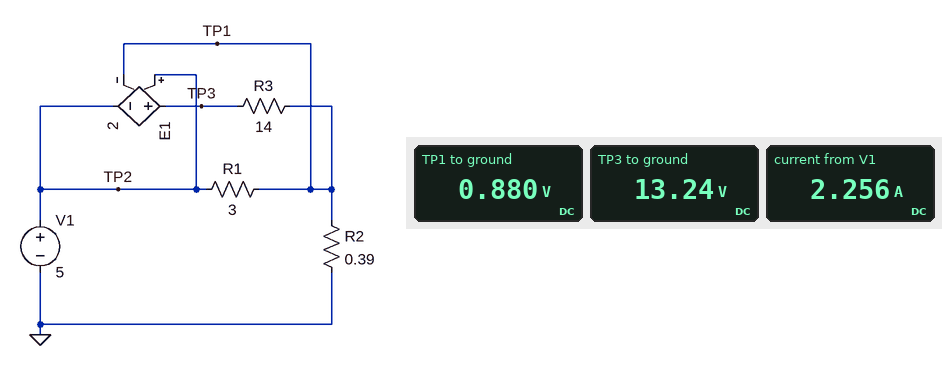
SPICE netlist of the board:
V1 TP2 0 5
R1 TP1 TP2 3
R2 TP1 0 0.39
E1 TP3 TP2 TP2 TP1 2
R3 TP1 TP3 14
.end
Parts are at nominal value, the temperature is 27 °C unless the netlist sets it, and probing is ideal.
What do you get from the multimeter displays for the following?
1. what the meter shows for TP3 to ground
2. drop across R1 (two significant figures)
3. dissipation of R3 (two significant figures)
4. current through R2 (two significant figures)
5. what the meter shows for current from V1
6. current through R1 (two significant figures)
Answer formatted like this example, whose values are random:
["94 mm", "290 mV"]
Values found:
["13.24 V", "4.1 V", "11 W", "2.3 A", "2.256 A", "1.4 A"]
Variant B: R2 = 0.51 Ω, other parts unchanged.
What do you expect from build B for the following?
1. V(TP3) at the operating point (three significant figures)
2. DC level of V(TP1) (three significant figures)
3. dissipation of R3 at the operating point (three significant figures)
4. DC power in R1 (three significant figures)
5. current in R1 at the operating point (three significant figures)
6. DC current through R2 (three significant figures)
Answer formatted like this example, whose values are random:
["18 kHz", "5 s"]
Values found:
["12.8 V", "1.09 V", "9.82 W", "5.09 W", "1.30 A", "2.14 A"]
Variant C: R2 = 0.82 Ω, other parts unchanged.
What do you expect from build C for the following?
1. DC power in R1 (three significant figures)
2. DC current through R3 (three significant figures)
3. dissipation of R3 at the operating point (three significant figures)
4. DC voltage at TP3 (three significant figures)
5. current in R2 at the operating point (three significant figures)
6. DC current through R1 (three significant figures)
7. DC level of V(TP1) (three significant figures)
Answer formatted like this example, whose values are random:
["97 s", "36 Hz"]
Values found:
["3.97 W", "739 mA", "7.65 W", "11.9 V", "1.89 A", "1.15 A", "1.55 V"]
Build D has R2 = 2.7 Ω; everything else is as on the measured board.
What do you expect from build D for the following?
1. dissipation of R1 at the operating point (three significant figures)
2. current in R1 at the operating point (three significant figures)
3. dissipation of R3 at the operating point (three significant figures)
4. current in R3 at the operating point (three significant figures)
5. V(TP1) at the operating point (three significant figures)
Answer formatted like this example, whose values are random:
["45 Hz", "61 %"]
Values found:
["1.36 W", "672 mA", "2.62 W", "432 mA", "2.98 V"]
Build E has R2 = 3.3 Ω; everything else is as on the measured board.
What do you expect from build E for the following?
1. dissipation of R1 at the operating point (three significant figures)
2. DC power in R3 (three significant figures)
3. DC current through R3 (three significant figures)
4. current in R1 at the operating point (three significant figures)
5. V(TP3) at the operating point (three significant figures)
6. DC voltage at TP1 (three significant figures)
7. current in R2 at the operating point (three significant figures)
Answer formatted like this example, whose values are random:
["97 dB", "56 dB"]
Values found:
["1.06 W", "2.04 W", "382 mA", "594 mA", "8.56 V", "3.22 V", "975 mA"]
